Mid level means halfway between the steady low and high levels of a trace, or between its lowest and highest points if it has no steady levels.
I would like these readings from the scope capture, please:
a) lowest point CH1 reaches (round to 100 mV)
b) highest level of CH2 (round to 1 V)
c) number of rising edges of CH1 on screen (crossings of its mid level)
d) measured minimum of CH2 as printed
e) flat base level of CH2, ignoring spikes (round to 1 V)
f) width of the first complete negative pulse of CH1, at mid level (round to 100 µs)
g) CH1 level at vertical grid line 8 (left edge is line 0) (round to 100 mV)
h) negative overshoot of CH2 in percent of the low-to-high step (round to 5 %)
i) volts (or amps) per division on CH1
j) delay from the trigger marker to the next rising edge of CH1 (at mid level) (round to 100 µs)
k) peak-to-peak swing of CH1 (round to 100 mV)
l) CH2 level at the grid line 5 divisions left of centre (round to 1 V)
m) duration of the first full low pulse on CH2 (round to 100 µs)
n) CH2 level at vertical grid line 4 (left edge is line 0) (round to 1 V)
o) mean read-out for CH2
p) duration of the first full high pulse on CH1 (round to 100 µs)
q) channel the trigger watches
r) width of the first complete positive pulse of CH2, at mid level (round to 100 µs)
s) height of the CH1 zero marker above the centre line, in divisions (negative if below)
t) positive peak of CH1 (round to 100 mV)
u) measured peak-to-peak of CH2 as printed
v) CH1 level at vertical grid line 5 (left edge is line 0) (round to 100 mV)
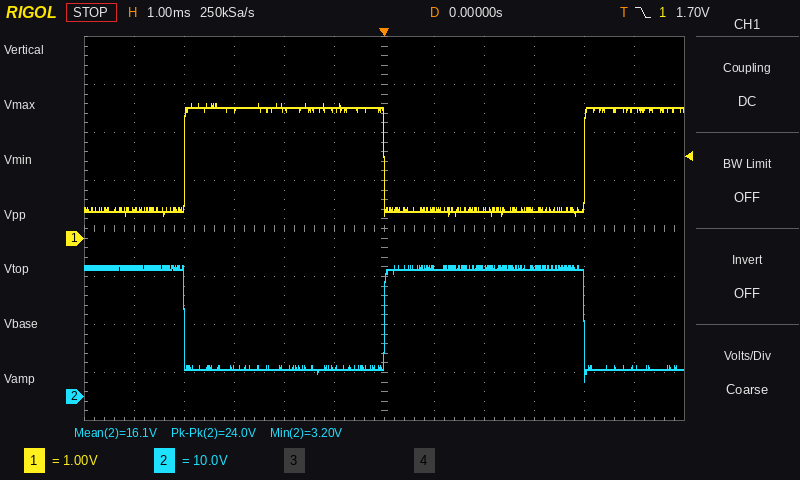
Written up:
500 mV
27 V
2
3.20 V
6 V
4.0 ms
600 mV
10 %
1 V
4.0 ms
2.3 V
27 V
4.0 ms
6 V
16.1 V
4.0 ms
CH1
4.0 ms
-0.2 div
2.8 V
24.0 V
2.7 V
